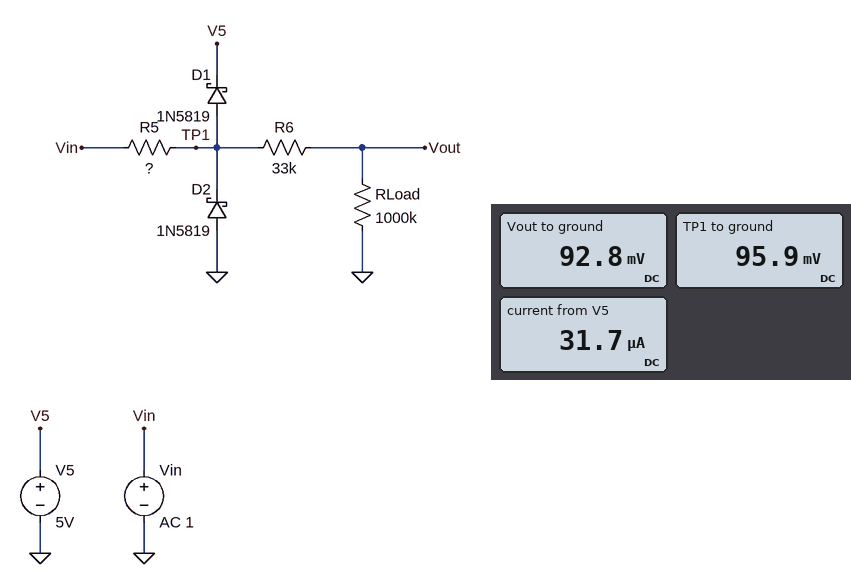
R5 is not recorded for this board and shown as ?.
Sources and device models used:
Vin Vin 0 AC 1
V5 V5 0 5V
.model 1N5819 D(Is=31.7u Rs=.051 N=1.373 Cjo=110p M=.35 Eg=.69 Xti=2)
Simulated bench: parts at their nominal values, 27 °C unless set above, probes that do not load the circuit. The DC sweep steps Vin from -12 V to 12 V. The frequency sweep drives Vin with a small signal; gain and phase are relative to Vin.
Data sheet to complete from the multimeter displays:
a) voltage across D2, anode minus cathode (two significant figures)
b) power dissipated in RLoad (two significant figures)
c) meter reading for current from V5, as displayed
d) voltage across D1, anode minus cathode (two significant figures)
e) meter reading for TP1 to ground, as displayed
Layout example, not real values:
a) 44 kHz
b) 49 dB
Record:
a) -96 mV
b) 8.6 nW
c) 31.7 µA
d) -4.9 V
e) 95.9 mV
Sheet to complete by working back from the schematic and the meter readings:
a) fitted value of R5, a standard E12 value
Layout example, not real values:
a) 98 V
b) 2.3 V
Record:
a) 47 kΩ
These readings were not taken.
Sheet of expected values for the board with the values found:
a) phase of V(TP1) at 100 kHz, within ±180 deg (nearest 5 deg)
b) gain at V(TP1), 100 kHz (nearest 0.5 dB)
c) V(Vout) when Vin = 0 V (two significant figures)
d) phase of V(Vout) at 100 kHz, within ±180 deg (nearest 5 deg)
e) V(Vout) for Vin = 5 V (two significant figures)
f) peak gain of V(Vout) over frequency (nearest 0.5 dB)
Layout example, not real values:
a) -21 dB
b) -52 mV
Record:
a) -50 deg
b) -16.0 dB
c) 93 mV
d) -50 deg
e) 4.6 V
f) -12.0 dB
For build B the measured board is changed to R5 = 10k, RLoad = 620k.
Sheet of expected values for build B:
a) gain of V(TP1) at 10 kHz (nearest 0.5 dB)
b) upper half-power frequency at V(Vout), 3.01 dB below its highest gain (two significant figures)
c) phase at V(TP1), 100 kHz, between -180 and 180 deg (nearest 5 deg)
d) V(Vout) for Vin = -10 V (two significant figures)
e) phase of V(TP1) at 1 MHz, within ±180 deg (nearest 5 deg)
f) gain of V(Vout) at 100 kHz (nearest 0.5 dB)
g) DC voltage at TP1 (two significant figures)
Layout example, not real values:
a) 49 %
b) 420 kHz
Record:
a) -8.5 dB
b) 260 kHz
c) -20 deg
d) -120 mV
e) -75 deg
f) -9.5 dB
g) 59 mV
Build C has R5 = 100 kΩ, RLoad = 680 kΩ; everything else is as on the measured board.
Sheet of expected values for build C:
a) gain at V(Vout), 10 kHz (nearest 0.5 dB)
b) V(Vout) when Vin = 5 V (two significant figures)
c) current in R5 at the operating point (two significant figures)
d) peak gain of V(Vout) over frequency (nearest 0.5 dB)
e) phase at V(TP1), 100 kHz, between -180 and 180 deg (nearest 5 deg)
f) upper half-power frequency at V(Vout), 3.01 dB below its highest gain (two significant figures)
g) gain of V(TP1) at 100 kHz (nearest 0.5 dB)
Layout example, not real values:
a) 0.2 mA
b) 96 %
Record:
a) -14.0 dB
b) 4.2 V
c) 1.1 µA
d) -13.5 dB
e) -65 deg
f) 44 kHz
g) -21.0 dB
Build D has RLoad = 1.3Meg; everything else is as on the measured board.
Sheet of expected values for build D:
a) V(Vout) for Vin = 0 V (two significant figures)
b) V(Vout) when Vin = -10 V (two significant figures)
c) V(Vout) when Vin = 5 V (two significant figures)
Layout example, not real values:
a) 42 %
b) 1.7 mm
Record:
a) 94 mV
b) -66 mV
c) 4.7 V
